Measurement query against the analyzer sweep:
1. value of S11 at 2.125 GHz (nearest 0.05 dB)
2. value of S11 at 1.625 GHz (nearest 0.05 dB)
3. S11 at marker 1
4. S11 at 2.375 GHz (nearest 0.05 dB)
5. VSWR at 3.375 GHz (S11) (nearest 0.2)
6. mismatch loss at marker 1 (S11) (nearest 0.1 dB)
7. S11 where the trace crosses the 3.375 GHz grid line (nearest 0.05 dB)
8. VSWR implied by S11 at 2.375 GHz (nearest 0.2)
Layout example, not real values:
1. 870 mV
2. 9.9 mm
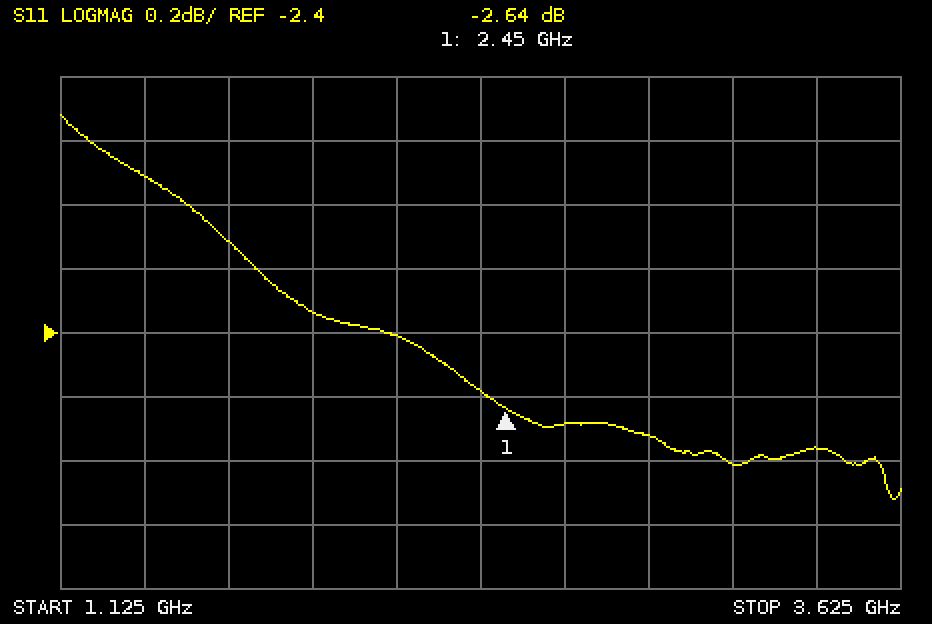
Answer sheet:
1. -2.40 dB
2. -2.10 dB
3. -2.64 dB
4. -2.60 dB
5. 6.4
6. 3.4 dB
7. -2.75 dB
8. 6.8
